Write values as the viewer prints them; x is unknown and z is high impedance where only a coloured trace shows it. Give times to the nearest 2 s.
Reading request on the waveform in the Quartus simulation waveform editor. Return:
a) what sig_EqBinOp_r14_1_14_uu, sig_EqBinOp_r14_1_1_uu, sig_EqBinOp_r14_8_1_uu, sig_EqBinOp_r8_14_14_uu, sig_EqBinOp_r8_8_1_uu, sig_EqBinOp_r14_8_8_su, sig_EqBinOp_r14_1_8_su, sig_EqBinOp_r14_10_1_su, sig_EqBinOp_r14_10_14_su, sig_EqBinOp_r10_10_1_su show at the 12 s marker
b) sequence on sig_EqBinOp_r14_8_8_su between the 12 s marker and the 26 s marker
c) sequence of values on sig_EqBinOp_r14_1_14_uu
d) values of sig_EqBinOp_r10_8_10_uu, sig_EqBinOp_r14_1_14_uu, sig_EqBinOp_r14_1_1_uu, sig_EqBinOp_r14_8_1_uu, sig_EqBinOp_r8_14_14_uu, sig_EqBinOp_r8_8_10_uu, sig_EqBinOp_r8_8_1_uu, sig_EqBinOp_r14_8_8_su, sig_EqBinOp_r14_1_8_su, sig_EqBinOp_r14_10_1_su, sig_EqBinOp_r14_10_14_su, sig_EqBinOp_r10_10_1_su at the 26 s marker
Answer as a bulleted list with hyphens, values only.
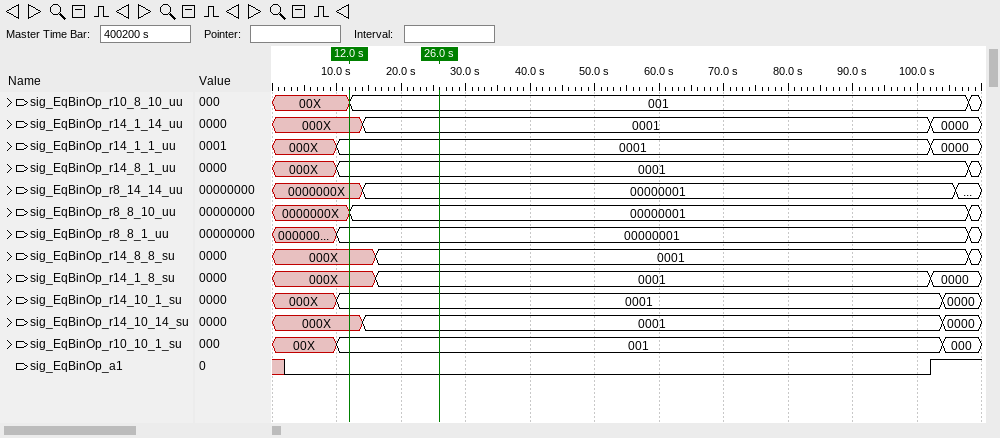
- sig_EqBinOp_r14_1_14_uu=000X, sig_EqBinOp_r14_1_1_uu=0001, sig_EqBinOp_r14_8_1_uu=0001, sig_EqBinOp_r8_14_14_uu=0000000X, sig_EqBinOp_r8_8_1_uu=00000001, sig_EqBinOp_r14_8_8_su=000X, sig_EqBinOp_r14_1_8_su=000X, sig_EqBinOp_r14_10_1_su=0001, sig_EqBinOp_r14_10_14_su=000X, sig_EqBinOp_r10_10_1_su=001
- 000X, 0001
- 000X, 0001, 0000
- sig_EqBinOp_r10_8_10_uu=001, sig_EqBinOp_r14_1_14_uu=0001, sig_EqBinOp_r14_1_1_uu=0001, sig_EqBinOp_r14_8_1_uu=0001, sig_EqBinOp_r8_14_14_uu=00000001, sig_EqBinOp_r8_8_10_uu=00000001, sig_EqBinOp_r8_8_1_uu=00000001, sig_EqBinOp_r14_8_8_su=0001, sig_EqBinOp_r14_1_8_su=0001, sig_EqBinOp_r14_10_1_su=0001, sig_EqBinOp_r14_10_14_su=0001, sig_EqBinOp_r10_10_1_su=001
